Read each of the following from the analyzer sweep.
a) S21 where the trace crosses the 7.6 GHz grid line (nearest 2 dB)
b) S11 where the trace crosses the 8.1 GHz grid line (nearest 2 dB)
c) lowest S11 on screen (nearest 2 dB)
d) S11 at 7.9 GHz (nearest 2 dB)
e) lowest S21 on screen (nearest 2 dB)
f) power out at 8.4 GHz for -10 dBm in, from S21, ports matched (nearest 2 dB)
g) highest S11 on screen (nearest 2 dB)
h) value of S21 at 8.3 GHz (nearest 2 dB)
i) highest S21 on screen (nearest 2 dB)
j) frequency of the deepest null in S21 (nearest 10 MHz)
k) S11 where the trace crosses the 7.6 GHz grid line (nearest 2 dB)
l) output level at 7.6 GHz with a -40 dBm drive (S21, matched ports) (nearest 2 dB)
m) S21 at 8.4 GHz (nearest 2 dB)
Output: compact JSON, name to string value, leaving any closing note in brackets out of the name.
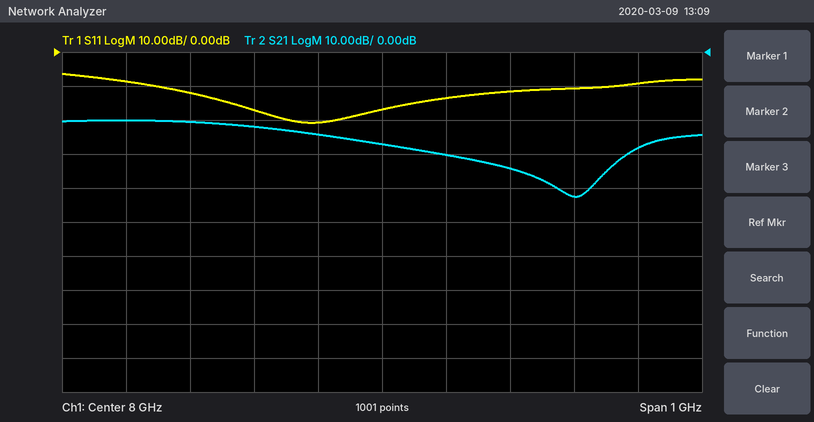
{"S21 where the trace crosses the 7.6 GHz grid line": "-20 dB", "S11 where the trace crosses the 8.1 GHz grid line": "-14 dB", "lowest S11 on screen": "-20 dB", "S11 at 7.9 GHz": "-20 dB", "lowest S21 on screen": "-42 dB", "power out at 8.4 GHz for -10 dBm in, from S21, ports matched": "-38 dBm", "highest S11 on screen": "-6 dB", "value of S21 at 8.3 GHz": "-42 dB", "highest S21 on screen": "-20 dB", "frequency of the deepest null in S21": "8.30 GHz", "S11 where the trace crosses the 7.6 GHz grid line": "-8 dB", "output level at 7.6 GHz with a -40 dBm drive (S21, matched ports)": "-60 dBm", "S21 at 8.4 GHz": "-28 dB"}
